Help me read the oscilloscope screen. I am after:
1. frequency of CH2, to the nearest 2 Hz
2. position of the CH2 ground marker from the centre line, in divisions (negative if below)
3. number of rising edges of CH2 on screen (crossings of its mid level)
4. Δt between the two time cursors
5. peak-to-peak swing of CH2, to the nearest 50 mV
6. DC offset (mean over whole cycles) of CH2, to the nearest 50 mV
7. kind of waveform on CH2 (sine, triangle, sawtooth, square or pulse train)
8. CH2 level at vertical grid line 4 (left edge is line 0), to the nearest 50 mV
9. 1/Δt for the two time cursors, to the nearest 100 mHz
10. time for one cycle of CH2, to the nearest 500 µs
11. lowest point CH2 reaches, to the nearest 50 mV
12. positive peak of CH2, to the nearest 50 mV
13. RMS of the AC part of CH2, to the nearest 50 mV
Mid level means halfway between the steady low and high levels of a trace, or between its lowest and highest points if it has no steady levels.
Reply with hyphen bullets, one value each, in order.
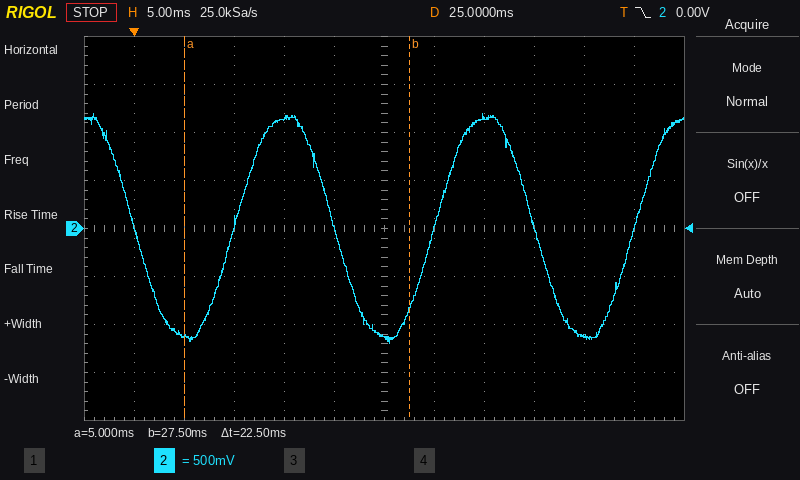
- 50 Hz
- 0.0 div
- 3
- 22.5 ms
- 2.40 V
- 0 mV
- sine
- 1.15 V
- 44.4 Hz
- 20.0 ms
- -1.20 V
- 1.20 V
- 850 mV
